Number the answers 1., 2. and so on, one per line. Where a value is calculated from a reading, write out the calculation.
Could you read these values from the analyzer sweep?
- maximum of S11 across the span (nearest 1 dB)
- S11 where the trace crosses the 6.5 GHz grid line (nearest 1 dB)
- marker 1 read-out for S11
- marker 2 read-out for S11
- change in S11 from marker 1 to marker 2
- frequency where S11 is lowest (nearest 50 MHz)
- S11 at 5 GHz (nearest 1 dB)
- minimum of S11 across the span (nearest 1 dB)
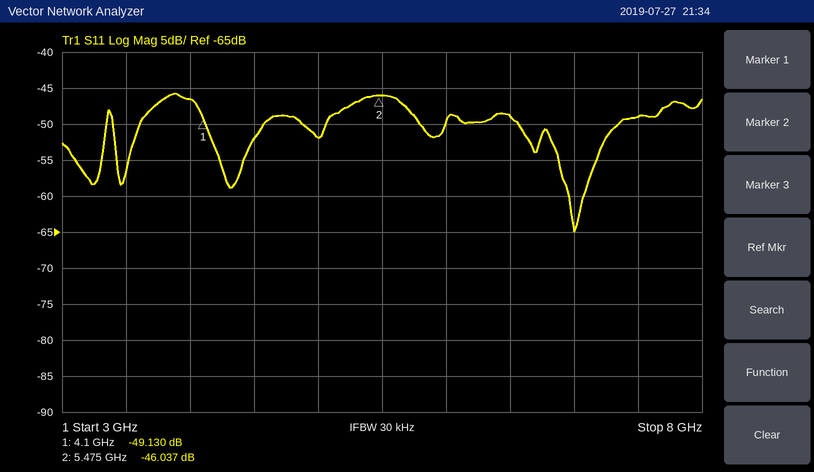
1. -46 dB
2. -49 dB
3. -49.130 dB
4. -46.037 dB
5. -46.037 − (-49.13) = 3.093 dB
6. 7.00 GHz
7. -52 dB
8. -65 dB
